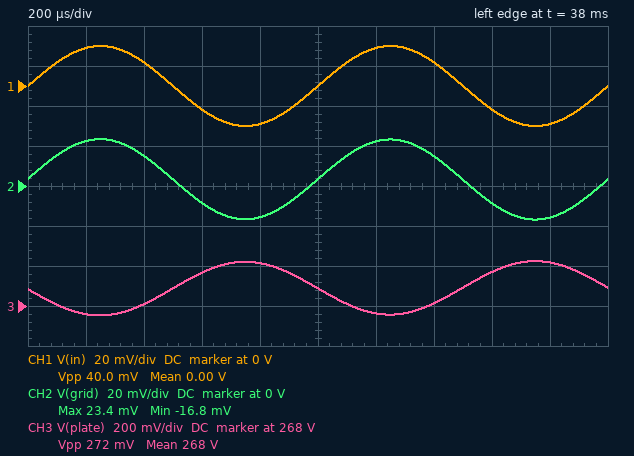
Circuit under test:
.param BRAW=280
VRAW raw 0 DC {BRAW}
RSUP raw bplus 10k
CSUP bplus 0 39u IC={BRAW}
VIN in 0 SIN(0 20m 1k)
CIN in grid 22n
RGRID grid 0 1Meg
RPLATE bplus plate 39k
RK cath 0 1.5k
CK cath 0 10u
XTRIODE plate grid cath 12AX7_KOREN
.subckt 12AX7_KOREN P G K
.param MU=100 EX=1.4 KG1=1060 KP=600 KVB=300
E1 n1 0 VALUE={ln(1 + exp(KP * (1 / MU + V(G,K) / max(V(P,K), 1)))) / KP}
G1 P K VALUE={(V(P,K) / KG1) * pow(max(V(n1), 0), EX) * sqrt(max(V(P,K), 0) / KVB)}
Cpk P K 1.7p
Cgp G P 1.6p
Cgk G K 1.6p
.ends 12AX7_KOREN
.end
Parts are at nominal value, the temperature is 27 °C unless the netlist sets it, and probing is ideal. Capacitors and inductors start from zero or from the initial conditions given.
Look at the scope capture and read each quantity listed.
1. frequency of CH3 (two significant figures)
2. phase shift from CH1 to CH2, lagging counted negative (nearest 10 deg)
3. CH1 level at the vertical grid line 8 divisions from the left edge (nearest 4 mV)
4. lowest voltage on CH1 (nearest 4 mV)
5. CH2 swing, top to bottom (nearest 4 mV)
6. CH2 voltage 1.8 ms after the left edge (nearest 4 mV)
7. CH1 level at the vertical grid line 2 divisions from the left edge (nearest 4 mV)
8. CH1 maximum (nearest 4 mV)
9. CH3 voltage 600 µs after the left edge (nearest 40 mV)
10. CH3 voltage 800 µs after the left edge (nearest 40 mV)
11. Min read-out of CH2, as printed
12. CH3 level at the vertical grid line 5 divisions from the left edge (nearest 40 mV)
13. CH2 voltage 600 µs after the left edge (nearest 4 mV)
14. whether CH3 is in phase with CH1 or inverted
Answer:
1.0 kHz
0 deg
-12 mV
-20 mV
40 mV
-16 mV
12 mV
20 mV
268.16 V
268.20 V
-16.8 mV
268.08 V
-8 mV
inverted
